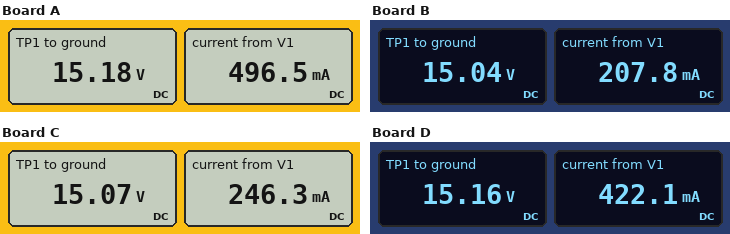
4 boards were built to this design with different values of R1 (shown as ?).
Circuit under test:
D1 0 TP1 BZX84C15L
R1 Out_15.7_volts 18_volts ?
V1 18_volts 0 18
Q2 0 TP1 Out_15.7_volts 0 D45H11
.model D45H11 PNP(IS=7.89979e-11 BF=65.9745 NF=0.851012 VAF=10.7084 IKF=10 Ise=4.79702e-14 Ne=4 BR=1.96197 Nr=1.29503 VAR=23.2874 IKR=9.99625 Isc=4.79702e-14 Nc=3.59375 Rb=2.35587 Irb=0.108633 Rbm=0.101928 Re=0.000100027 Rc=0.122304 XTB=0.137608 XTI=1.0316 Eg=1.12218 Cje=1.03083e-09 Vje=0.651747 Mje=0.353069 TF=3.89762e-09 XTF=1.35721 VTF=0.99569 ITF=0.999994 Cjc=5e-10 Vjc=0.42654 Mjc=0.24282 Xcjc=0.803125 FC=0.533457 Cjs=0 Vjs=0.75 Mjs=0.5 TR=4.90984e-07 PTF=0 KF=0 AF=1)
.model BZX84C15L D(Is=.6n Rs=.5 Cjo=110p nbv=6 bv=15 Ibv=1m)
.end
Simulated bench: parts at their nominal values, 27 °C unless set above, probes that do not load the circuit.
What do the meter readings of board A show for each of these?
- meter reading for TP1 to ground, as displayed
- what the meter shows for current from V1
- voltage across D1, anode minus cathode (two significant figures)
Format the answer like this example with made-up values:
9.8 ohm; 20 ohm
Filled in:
15.18 V; 496.5 mA; -15 V
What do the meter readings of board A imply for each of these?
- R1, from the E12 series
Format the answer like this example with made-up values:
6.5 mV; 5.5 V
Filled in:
4.7 Ω
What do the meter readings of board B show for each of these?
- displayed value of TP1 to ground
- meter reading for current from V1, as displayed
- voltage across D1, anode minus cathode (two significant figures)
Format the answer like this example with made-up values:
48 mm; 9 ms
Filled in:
15.04 V; 207.8 mA; -15 V
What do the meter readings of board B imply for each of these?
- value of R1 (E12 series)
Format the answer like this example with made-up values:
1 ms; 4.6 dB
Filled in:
12 Ω
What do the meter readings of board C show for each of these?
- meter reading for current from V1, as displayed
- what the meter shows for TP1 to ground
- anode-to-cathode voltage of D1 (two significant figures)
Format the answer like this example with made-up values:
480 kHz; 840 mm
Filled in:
246.3 mA; 15.07 V; -15 V
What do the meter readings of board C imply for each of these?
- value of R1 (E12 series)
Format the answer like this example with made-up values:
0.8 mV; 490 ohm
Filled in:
10 Ω
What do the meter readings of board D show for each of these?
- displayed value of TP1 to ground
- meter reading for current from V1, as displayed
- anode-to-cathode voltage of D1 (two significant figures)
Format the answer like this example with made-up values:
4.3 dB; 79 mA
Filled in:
15.16 V; 422.1 mA; -15 V
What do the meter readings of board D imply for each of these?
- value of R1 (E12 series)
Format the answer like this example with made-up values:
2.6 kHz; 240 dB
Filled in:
5.6 Ω
